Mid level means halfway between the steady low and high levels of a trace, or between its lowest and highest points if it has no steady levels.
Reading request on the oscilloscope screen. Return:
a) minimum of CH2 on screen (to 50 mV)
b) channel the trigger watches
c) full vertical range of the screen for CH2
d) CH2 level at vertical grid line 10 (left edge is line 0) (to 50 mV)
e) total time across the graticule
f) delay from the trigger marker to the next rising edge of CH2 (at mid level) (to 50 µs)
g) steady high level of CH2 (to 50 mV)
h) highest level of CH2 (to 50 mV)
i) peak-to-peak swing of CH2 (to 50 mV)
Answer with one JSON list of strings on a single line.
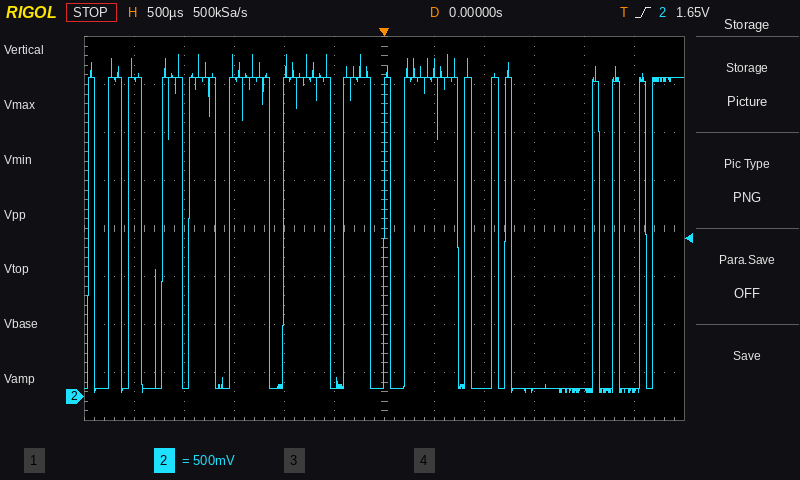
["50 mV", "CH2", "4 V", "50 mV", "6 ms", "200 µs", "3.30 V", "3.55 V", "3.50 V"]
